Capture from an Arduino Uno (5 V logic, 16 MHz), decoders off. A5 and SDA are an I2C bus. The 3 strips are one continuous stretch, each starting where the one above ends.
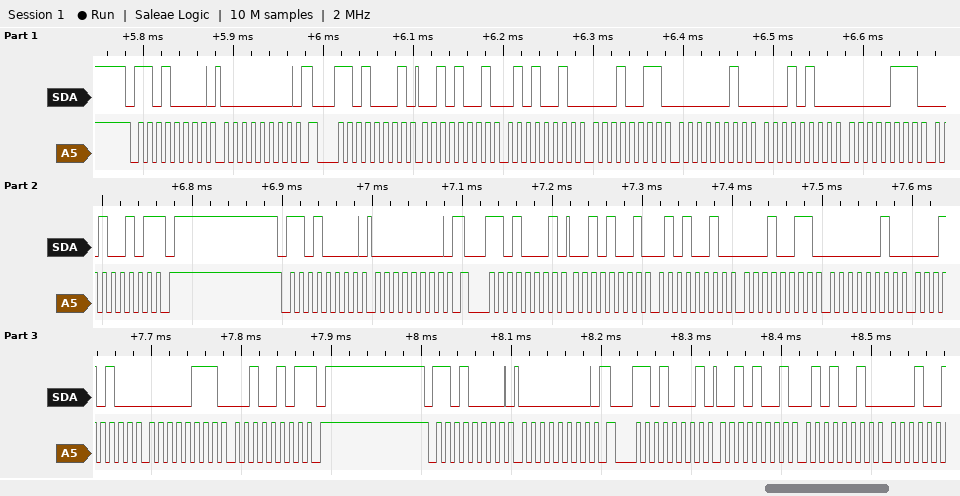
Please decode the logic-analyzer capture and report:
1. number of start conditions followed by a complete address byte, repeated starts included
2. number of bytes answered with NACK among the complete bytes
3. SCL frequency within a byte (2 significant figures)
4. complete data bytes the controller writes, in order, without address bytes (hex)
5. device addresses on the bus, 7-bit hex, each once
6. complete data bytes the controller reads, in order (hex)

6
2
100 kHz
00 00 00
0x68
29 52 13 02 14 07 25 29 52 13 02 14 07 25 29 52
